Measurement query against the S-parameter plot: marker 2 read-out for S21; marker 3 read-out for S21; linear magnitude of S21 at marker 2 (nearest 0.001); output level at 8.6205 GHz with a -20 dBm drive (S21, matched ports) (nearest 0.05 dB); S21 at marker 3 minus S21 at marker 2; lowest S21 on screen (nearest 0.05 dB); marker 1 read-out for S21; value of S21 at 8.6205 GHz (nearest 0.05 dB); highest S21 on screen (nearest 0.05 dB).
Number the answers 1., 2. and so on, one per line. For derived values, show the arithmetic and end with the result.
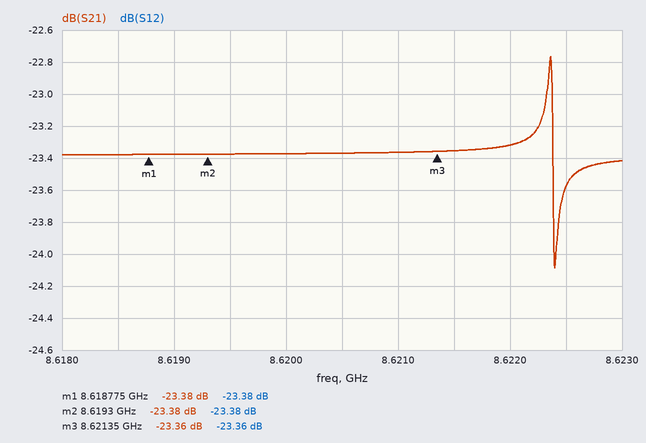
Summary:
1. -23.38 dB
2. -23.36 dB
3. 10^(-23.38/20) ≈ 0.068
4. -20 dBm + (-23.35 dB) = -43.35 dBm
5. -23.36 − (-23.38) = 0.02 dB
6. -24.10 dB
7. -23.38 dB
8. -23.35 dB
9. -22.75 dB
